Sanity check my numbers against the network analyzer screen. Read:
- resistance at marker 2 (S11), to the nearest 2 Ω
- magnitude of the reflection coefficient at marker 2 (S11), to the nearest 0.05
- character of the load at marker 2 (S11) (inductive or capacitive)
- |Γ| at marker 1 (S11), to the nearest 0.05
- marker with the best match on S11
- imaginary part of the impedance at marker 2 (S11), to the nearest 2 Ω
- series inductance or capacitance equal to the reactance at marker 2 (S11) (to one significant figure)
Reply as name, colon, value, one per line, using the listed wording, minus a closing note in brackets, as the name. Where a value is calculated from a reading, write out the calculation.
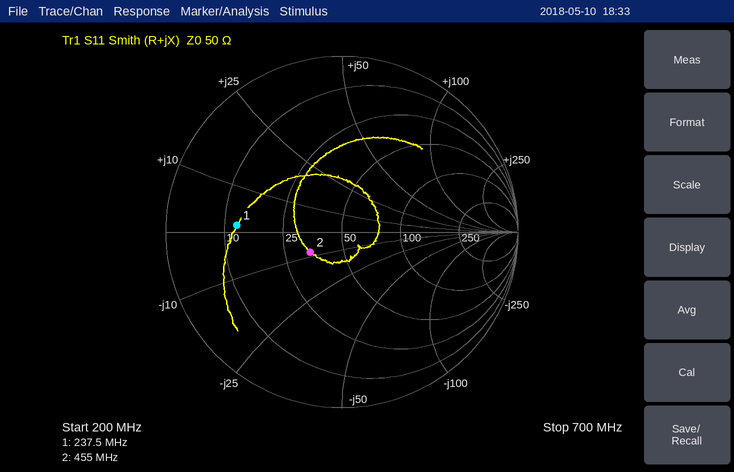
resistance at marker 2 (S11), to the nearest 2 Ω: 34 Ω
magnitude of the reflection coefficient at marker 2 (S11), to the nearest 0.05: 0.20
character of the load at marker 2 (S11): capacitive
|Γ| at marker 1 (S11), to the nearest 0.05: 0.60
marker with the best match on S11: marker 2
imaginary part of the impedance at marker 2 (S11), to the nearest 2 Ω: -8 Ω
series inductance or capacitance equal to the reactance at marker 2 (S11): C = 1/(2π × 455 MHz × 8 Ω) ≈ 43.7 pF, so 40 pF to one significant figure
